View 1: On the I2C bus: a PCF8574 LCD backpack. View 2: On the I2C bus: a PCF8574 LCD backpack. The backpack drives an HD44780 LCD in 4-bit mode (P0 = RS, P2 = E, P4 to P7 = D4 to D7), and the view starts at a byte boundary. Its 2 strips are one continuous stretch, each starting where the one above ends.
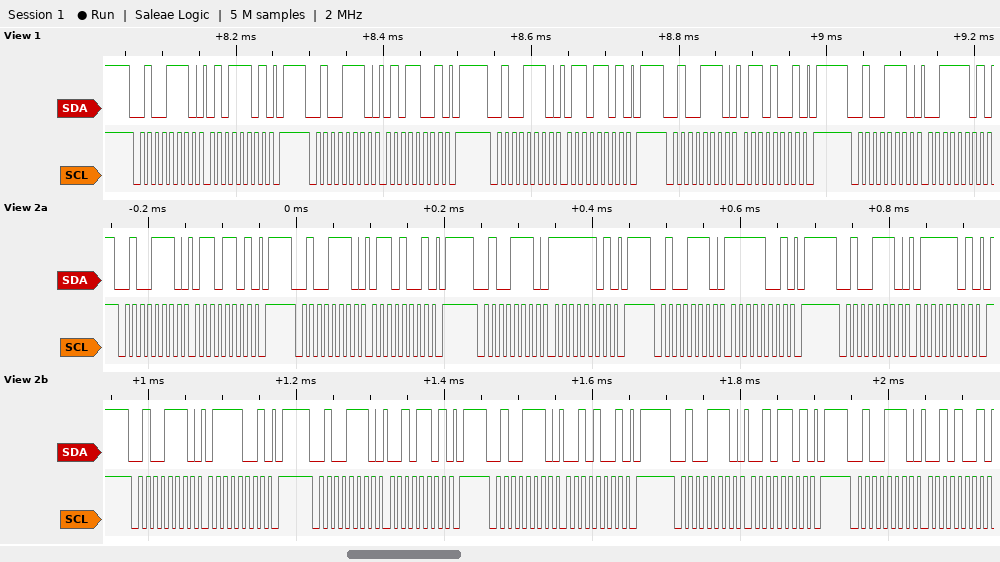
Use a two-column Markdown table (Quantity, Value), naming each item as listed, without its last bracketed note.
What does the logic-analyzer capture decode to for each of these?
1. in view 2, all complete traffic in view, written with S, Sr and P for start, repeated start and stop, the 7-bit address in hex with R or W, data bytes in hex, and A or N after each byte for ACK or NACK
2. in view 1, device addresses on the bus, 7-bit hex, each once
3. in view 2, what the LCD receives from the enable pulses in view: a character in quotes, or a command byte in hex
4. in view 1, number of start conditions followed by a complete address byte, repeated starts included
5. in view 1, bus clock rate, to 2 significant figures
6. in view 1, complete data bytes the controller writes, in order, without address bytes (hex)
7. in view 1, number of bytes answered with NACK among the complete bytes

| Quantity | Value |
|---|---|
| in view 2, all complete traffic in view, written with S, Sr and P for start, repeated start and stop, the 7-bit address in hex with R or W, data bytes in hex, and A or N after each byte for ACK or NACK | S 27W A 6D A P S 27W A 69 A P S 27W A FD A P S 27W A F9 A P S 27W A 7D A P S 27W A 79 A P S 27W A 2D A P S 27W A 29 A P S 27W A 2D A P S 27W A 29 A |
| in view 1, device addresses on the bus, 7-bit hex, each once | 0x27 |
| in view 2, what the LCD receives from the enable pulses in view: a character in quotes, or a command byte in hex | 'o' 'r' |
| in view 1, number of start conditions followed by a complete address byte, repeated starts included | 5 |
| in view 1, bus clock rate, to 2 significant figures | 100 kHz |
| in view 1, complete data bytes the controller writes, in order, without address bytes | 5D 59 6D 69 3D |
| in view 1, number of bytes answered with NACK among the complete bytes | 0 |
